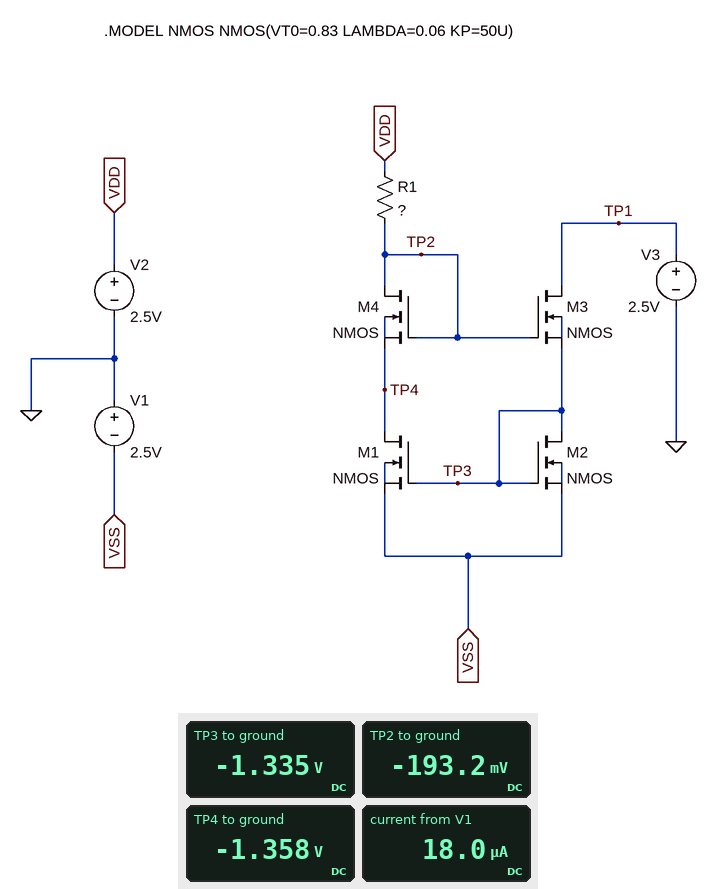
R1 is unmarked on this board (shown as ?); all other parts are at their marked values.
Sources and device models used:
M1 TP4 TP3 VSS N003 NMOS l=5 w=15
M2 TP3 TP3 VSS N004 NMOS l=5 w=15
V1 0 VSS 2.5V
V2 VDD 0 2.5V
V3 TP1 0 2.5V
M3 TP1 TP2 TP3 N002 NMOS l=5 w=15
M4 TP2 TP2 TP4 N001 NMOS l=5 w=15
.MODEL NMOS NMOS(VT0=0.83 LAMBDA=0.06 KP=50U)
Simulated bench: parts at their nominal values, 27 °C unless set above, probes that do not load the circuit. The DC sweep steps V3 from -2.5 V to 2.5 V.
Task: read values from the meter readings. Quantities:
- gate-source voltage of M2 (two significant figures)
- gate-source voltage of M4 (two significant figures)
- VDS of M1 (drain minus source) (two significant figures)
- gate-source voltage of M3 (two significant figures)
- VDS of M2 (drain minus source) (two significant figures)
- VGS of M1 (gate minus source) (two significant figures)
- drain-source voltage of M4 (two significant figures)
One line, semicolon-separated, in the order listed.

1.2 V; 1.2 V; 1.1 V; 1.1 V; 1.2 V; 1.2 V; 1.2 V
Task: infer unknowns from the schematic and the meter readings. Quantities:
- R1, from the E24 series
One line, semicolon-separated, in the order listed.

300 kΩ
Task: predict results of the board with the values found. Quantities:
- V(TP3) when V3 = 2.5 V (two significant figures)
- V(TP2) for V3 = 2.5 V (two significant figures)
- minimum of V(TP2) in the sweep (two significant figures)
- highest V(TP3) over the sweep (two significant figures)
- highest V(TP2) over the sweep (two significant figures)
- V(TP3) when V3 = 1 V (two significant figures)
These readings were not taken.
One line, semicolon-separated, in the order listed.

-1.3 V; -190 mV; -190 mV; -1.3 V; 2.5 V; -1.3 V
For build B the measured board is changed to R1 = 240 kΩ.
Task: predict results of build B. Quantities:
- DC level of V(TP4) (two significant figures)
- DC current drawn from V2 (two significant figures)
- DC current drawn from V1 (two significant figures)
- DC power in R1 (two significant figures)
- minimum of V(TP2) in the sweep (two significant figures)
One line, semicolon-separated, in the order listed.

-1.3 V; 11 µA; 22 µA; 29 µW; -130 mV
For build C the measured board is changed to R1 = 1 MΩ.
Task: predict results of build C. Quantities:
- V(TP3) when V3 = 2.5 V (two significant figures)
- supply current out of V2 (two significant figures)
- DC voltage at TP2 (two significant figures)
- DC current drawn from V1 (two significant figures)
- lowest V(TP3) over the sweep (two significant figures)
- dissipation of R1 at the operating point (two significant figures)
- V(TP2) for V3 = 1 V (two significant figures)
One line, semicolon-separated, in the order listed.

-1.5 V; 3.0 µA; -470 mV; 5.9 µA; -2.5 V; 8.8 µW; -460 mV
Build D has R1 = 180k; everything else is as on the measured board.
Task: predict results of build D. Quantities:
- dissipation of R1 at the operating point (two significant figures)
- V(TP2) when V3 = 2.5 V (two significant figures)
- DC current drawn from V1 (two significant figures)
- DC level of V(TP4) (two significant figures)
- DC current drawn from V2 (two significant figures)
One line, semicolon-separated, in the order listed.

36 µW; -31 mV; 28 µA; -1.3 V; 14 µA
